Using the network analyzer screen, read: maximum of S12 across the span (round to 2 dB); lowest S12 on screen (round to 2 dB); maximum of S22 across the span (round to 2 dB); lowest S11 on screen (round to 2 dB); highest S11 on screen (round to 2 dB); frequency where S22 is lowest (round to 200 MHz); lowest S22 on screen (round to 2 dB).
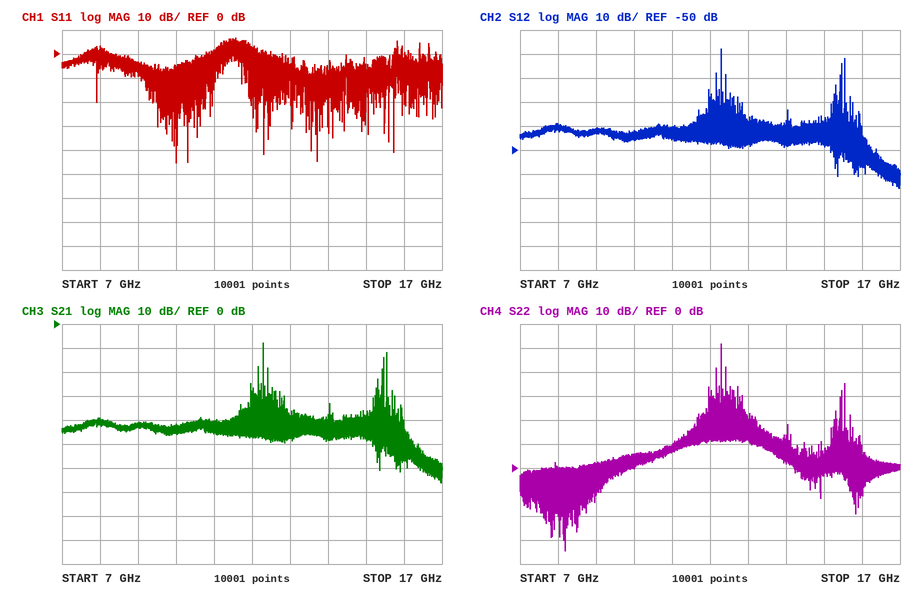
-8 dB
-66 dB
52 dB
-46 dB
6 dB
8.2 GHz
-34 dB
